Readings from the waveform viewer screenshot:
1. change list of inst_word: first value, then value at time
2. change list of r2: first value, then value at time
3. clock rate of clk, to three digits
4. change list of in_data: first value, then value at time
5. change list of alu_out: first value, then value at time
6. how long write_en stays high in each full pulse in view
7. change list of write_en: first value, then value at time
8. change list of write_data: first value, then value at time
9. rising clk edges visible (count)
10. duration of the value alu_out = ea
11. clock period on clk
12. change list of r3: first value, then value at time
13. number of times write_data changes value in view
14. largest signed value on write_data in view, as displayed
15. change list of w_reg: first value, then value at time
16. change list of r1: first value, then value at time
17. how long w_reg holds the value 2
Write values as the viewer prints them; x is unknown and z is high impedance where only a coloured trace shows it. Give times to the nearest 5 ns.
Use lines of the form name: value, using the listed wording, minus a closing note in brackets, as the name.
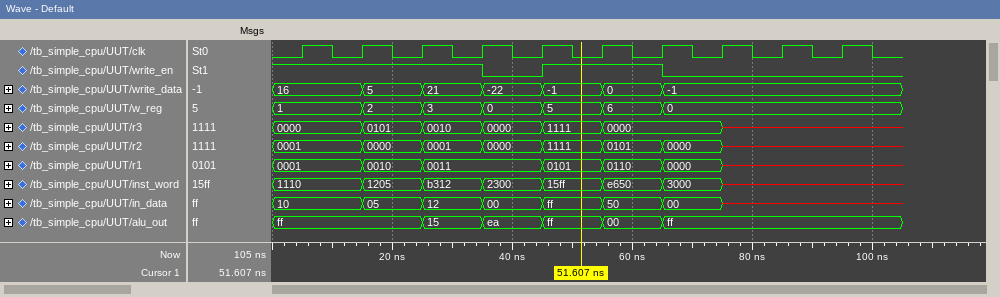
change list of inst_word: first value, then value at time: 1110, 1205 at 15 ns, b312 at 25 ns, 2300 at 35 ns, 15ff at 45 ns, e650 at 55 ns, 3000 at 65 ns, x at 75 ns
change list of r2: first value, then value at time: 0001, 0000 at 15 ns, 0001 at 25 ns, 0000 at 35 ns, 1111 at 45 ns, 0101 at 55 ns, 0000 at 65 ns, x at 75 ns
clock rate of clk, to three digits: 100 MHz
change list of in_data: first value, then value at time: 10, 05 at 15 ns, 12 at 25 ns, 00 at 35 ns, ff at 45 ns, 50 at 55 ns, 00 at 65 ns, x at 75 ns
change list of alu_out: first value, then value at time: ff, 15 at 25 ns, ea at 35 ns, ff at 45 ns, 00 at 55 ns, ff at 65 ns
how long write_en stays high in each full pulse in view: 20 ns
change list of write_en: first value, then value at time: 1, 0 at 35 ns, 1 at 45 ns, 0 at 65 ns
change list of write_data: first value, then value at time: 16, 5 at 15 ns, 21 at 25 ns, -22 at 35 ns, -1 at 45 ns, 0 at 55 ns, -1 at 65 ns
rising clk edges visible: 10
duration of the value alu_out = ea: 10 ns
clock period on clk: 10 ns
change list of r3: first value, then value at time: 0000, 0101 at 15 ns, 0010 at 25 ns, 0000 at 35 ns, 1111 at 45 ns, 0000 at 55 ns, x at 75 ns
number of times write_data changes value in view: 6
largest signed value on write_data in view, as displayed: 21
change list of w_reg: first value, then value at time: 1, 2 at 15 ns, 3 at 25 ns, 0 at 35 ns, 5 at 45 ns, 6 at 55 ns, 0 at 65 ns
change list of r1: first value, then value at time: 0001, 0010 at 15 ns, 0011 at 25 ns, 0101 at 45 ns, 0110 at 55 ns, 0000 at 65 ns, x at 75 ns
how long w_reg holds the value 2: 10 ns
